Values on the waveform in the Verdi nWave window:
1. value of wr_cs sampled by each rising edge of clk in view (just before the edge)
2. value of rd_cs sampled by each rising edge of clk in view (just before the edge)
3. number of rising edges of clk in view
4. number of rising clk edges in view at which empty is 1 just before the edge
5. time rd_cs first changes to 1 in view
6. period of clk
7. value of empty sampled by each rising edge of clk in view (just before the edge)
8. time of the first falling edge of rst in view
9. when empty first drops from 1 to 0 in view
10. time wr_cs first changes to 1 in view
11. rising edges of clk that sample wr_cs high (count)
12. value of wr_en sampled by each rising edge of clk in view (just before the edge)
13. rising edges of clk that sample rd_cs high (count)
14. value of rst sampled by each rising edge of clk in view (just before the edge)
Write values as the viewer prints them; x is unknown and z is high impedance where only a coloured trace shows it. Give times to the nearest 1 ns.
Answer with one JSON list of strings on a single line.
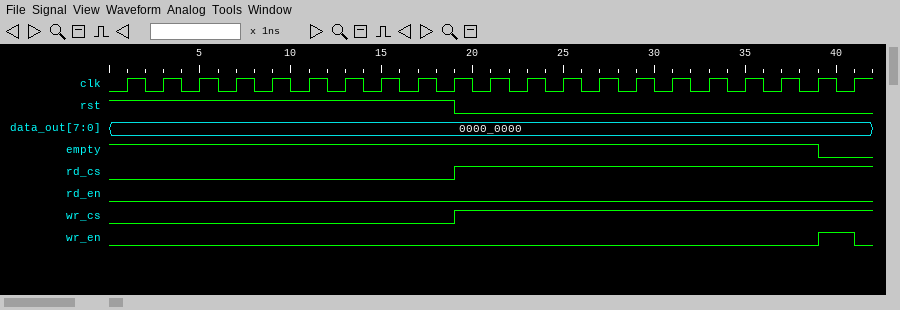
["0 0 0 0 0 0 0 0 0 0 1 1 1 1 1 1 1 1 1 1 1", "0 0 0 0 0 0 0 0 0 0 1 1 1 1 1 1 1 1 1 1 1", "21", "20", "19 ns", "2 ns", "1 1 1 1 1 1 1 1 1 1 1 1 1 1 1 1 1 1 1 1 0", "19 ns", "39 ns", "19 ns", "11", "0 0 0 0 0 0 0 0 0 0 0 0 0 0 0 0 0 0 0 0 1", "11", "1 1 1 1 1 1 1 1 1 1 0 0 0 0 0 0 0 0 0 0 0"]
